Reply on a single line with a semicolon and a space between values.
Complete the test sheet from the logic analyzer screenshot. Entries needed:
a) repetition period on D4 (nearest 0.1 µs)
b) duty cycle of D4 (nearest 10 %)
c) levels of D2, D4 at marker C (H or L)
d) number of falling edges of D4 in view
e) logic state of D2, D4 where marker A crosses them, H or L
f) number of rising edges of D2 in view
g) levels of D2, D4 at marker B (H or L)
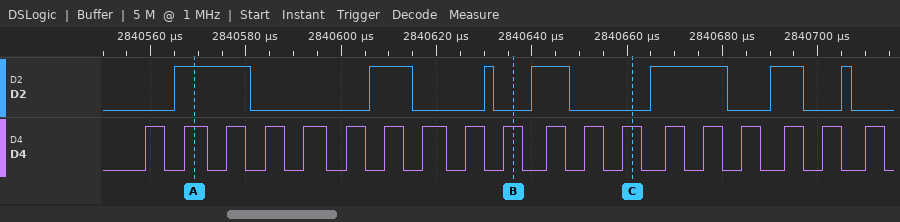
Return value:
8.4 µs; 50 %; D2=L, D4=H; 19; D2=H, D4=H; 7; D2=L, D4=H
